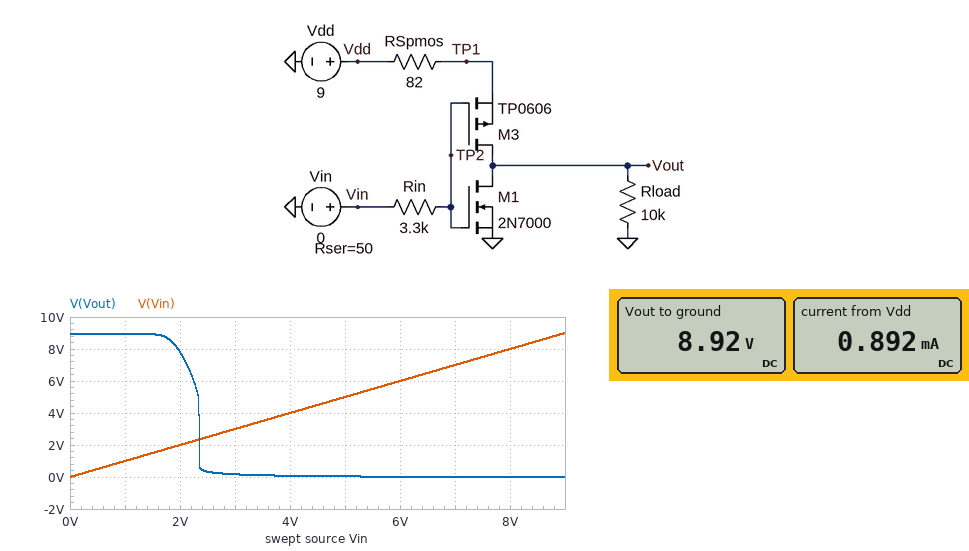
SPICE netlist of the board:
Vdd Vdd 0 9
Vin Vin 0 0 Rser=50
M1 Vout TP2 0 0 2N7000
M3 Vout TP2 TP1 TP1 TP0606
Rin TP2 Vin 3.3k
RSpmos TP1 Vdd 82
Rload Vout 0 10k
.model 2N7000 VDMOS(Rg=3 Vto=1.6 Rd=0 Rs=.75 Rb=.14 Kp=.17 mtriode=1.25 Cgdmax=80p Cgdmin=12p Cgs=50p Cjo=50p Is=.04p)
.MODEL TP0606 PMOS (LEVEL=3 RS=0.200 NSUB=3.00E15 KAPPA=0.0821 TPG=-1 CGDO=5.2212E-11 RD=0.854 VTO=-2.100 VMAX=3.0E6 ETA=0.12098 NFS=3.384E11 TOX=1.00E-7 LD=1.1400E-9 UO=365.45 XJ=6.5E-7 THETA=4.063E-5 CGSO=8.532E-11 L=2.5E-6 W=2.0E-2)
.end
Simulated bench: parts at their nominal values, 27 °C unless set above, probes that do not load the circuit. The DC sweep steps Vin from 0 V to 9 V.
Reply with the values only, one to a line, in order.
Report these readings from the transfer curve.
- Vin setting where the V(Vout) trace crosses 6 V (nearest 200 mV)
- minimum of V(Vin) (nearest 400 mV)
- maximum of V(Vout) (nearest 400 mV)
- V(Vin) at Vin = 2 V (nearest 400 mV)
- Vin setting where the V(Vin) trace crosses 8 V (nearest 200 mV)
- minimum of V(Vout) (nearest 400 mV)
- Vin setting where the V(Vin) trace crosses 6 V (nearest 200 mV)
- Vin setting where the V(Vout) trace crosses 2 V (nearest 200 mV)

2.2 V
0 V
8.8 V
2.0 V
8.0 V
0 V
6.0 V
2.4 V
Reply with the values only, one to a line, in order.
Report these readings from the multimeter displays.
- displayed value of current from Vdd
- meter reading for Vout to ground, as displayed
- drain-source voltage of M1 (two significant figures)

0.892 mA
8.92 V
8.9 V
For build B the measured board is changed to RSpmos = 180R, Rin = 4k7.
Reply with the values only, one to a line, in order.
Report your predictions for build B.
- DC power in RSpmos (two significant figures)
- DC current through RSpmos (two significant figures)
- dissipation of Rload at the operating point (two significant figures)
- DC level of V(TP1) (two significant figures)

140 µW
880 µA
7.8 mW
8.8 V
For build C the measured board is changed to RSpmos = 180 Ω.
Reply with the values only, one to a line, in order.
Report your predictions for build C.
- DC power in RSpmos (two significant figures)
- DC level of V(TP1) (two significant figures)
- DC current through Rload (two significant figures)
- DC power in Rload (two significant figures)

140 µW
8.8 V
880 µA
7.8 mW
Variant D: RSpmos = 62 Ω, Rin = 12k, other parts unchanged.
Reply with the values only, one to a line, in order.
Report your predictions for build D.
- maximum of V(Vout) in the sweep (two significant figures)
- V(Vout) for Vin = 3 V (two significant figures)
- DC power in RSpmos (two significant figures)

8.9 V
220 mV
50 µW
